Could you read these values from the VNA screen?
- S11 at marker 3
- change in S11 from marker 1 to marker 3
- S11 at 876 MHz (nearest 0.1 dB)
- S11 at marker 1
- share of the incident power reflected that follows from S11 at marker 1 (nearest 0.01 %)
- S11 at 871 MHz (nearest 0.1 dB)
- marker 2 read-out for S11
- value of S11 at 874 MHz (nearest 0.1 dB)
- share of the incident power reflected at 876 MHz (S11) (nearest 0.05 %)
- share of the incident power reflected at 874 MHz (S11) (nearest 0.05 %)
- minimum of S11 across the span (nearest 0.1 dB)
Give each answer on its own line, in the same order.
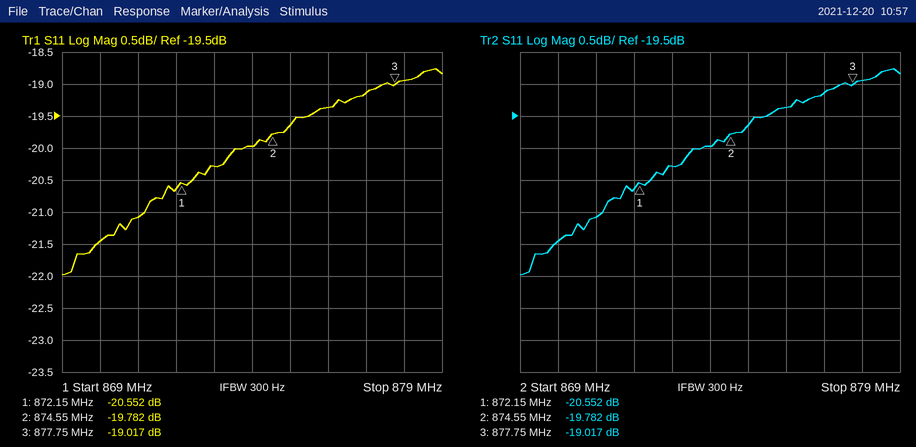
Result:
-19.017 dB
1.535 dB
-19.4 dB
-20.552 dB
0.88 %
-21.1 dB
-19.782 dB
-20.0 dB
1.15 %
1.00 %
-22.0 dB
